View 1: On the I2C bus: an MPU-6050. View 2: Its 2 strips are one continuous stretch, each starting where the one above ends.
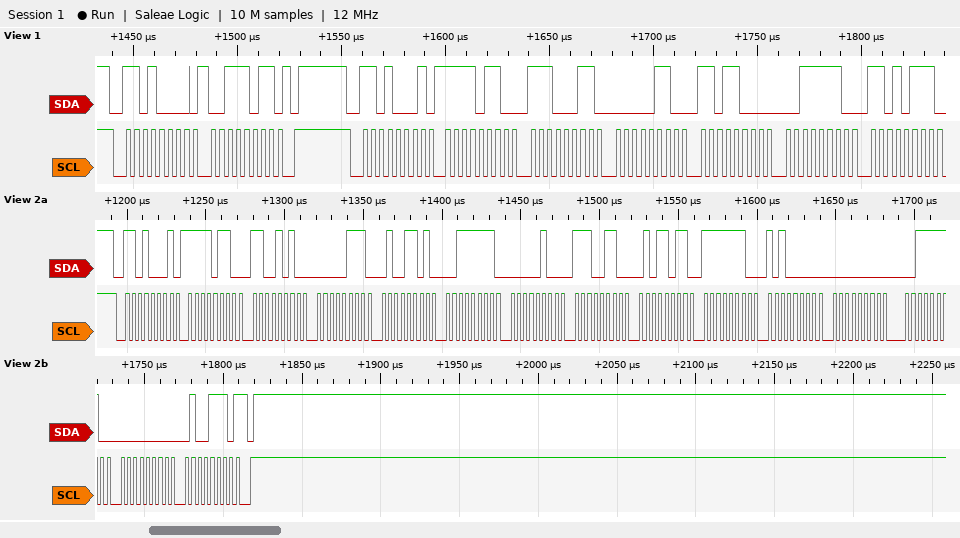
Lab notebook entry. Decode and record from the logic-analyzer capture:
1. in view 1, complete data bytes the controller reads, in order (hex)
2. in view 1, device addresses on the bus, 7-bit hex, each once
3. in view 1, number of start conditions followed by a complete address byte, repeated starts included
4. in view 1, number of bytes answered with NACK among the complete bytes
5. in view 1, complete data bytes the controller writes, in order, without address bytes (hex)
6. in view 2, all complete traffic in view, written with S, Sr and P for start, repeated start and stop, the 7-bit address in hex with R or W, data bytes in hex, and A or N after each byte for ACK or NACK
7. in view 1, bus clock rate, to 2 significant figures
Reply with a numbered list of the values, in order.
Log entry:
1. F6 E3 06 D8 3E D7
2. 0x68
3. 2
4. 0
5. 3B
6. S 68R A F6 A CA A 07 A 4D A 3F A 04 A E6 A 5B A FE A A0 A 00 A 3E A 00 A 4E N P
7. 250 kHz
